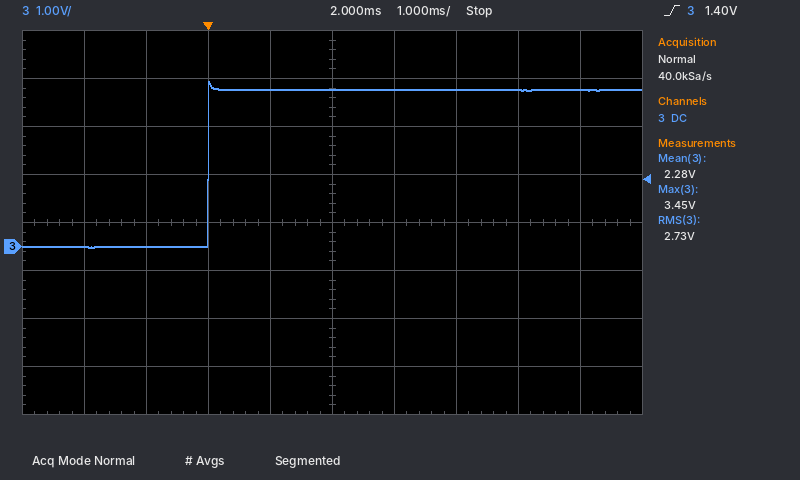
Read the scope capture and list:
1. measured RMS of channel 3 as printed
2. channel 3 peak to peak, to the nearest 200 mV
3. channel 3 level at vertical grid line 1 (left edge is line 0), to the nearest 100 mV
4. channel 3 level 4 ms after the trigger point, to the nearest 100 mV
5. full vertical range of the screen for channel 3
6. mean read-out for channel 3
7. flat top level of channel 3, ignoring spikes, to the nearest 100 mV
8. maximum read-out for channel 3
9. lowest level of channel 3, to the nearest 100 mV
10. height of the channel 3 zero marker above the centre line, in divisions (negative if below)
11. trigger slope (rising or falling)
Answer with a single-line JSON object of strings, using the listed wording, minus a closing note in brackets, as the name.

{"measured RMS of channel 3 as printed": "2.73 V", "channel 3 peak to peak, to the nearest 200 mV": "3.4 V", "channel 3 level at vertical grid line 1 (left edge is line 0), to the nearest 100 mV": "0.0 V", "channel 3 level 4 ms after the trigger point, to the nearest 100 mV": "3.3 V", "full vertical range of the screen for channel 3": "8 V", "mean read-out for channel 3": "2.28 V", "flat top level of channel 3, ignoring spikes, to the nearest 100 mV": "3.3 V", "maximum read-out for channel 3": "3.45 V", "lowest level of channel 3, to the nearest 100 mV": "0.0 V", "height of the channel 3 zero marker above the centre line, in divisions": "-0.5 div", "trigger slope": "rising"}
